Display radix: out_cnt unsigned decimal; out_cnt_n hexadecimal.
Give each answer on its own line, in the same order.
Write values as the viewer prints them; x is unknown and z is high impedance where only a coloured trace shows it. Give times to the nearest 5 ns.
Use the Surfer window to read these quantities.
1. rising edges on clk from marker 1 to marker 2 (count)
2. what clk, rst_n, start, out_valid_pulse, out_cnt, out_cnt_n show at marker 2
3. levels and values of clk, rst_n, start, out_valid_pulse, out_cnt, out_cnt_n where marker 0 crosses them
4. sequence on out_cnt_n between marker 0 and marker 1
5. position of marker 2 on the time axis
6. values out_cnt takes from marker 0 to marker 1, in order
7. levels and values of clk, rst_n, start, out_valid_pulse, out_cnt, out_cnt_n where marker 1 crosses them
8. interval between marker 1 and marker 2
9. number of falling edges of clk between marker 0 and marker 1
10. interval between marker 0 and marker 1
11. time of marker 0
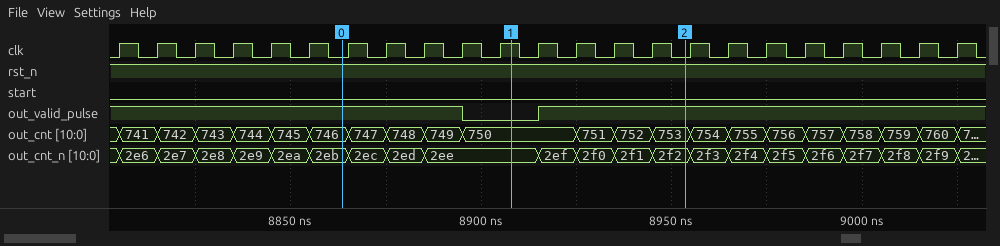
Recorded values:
4
clk=0, rst_n=1, start=0, out_valid_pulse=1, out_cnt=753, out_cnt_n=2f2
clk=0, rst_n=1, start=0, out_valid_pulse=1, out_cnt=746, out_cnt_n=2eb
2eb, 2ec, 2ed, 2ee
8955 ns
746, 747, 748, 749, 750
clk=1, rst_n=1, start=0, out_valid_pulse=0, out_cnt=750, out_cnt_n=2ee
45 ns
4
45 ns
8865 ns
